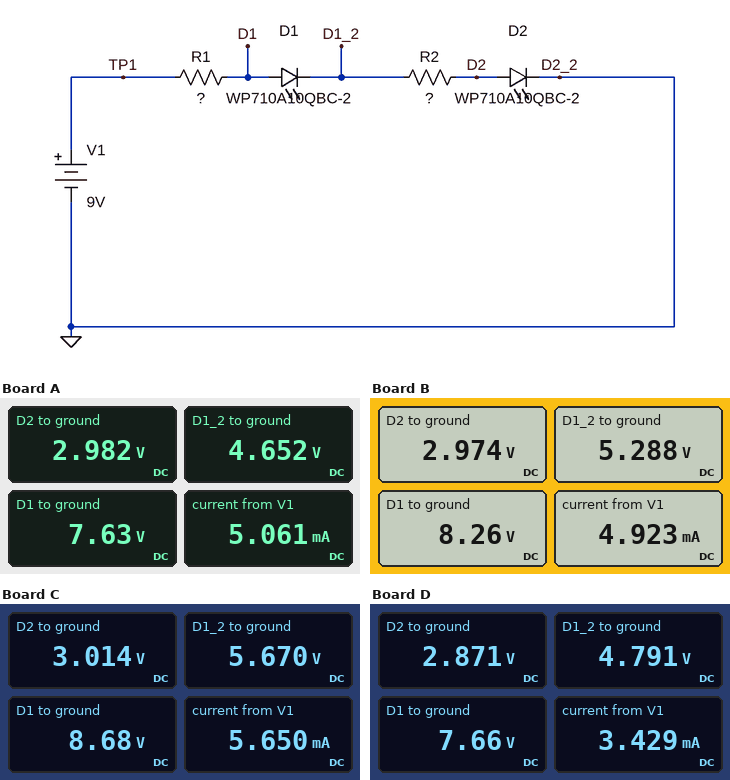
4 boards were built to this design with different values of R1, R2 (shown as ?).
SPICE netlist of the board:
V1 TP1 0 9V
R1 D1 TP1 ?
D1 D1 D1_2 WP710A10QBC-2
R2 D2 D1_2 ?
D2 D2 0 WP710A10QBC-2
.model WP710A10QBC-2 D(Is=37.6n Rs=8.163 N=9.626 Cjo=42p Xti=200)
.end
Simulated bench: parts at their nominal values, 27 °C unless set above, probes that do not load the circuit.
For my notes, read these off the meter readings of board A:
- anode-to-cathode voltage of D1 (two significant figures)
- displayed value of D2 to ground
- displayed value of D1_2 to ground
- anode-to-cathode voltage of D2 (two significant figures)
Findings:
3.0 V
2.982 V
4.652 V
3.0 V
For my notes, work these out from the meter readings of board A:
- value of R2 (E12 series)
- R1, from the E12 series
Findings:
330 Ω
270 Ω
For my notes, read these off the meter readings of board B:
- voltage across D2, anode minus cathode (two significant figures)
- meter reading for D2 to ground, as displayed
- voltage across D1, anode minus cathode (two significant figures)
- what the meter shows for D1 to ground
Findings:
3.0 V
2.974 V
3.0 V
8.26 V
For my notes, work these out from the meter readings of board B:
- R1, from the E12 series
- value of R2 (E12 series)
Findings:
150 Ω
470 Ω
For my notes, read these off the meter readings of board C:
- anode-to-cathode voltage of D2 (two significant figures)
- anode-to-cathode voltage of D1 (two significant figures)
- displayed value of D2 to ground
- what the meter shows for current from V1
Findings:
3.0 V
3.0 V
3.014 V
5.650 mA
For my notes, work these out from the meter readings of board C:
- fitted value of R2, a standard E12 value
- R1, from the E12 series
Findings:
470 Ω
56 Ω
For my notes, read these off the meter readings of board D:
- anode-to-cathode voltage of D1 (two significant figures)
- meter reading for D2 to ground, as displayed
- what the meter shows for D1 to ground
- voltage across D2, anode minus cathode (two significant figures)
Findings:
2.9 V
2.871 V
7.66 V
2.9 V
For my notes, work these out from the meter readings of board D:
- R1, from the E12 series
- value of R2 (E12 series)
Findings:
390 Ω
560 Ω
